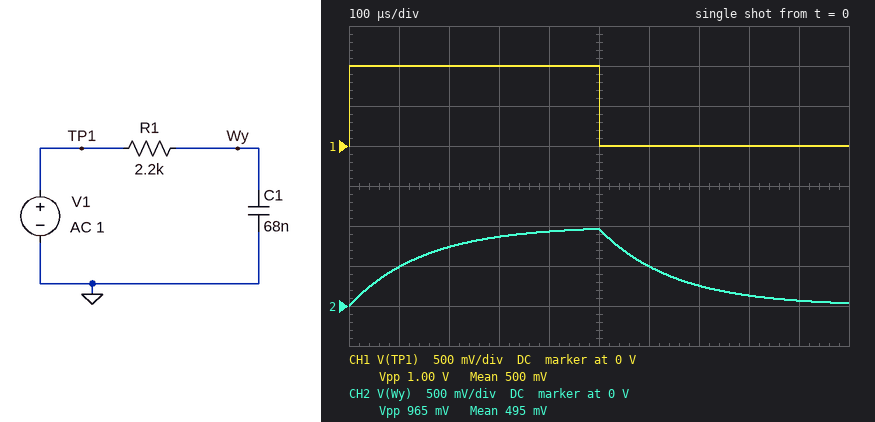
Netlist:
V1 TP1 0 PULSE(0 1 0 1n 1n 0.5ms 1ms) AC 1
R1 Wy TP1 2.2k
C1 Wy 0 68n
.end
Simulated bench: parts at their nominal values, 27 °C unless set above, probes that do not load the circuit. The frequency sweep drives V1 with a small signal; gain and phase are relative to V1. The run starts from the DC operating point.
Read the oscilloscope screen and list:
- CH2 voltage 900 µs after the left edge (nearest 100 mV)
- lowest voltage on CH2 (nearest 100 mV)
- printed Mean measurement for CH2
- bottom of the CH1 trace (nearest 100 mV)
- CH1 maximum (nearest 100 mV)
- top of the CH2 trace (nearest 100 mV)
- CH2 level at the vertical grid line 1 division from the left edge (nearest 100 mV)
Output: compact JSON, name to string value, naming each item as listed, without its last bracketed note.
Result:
{"CH2 voltage 900 µs after the left edge": "100 mV", "lowest voltage on CH2": "0 V", "printed Mean measurement for CH2": "495 mV", "bottom of the CH1 trace": "0 V", "CH1 maximum": "1.0 V", "top of the CH2 trace": "1.0 V", "CH2 level at the vertical grid line 1 division from the left edge": "500 mV"}
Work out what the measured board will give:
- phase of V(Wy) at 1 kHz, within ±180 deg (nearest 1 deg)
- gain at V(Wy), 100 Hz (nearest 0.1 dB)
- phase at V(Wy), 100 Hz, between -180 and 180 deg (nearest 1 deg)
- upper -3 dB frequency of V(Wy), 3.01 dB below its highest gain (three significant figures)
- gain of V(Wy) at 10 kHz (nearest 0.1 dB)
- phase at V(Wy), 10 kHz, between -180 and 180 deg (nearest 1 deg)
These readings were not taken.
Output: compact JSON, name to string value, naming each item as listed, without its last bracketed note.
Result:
{"phase of V(Wy) at 1 kHz, within ±180 deg": "-43 deg", "gain at V(Wy), 100 Hz": "0 dB", "phase at V(Wy), 100 Hz, between -180 and 180 deg": "-5 deg", "upper -3 dB frequency of V(Wy), 3.01 dB below its highest gain": "1.06 kHz", "gain of V(Wy) at 10 kHz": "-19.5 dB", "phase at V(Wy), 10 kHz, between -180 and 180 deg": "-84 deg"}
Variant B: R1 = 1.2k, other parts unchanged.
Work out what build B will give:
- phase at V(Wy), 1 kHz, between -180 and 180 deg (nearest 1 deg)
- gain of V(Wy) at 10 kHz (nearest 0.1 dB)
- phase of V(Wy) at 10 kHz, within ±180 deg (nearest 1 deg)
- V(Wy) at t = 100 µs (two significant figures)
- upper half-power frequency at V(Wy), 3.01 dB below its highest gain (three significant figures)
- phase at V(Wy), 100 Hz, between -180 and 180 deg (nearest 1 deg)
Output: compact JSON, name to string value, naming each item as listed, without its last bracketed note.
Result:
{"phase at V(Wy), 1 kHz, between -180 and 180 deg": "-27 deg", "gain of V(Wy) at 10 kHz": "-14.4 dB", "phase of V(Wy) at 10 kHz, within ±180 deg": "-79 deg", "V(Wy) at t = 100 µs": "710 mV", "upper half-power frequency at V(Wy), 3.01 dB below its highest gain": "1.95 kHz", "phase at V(Wy), 100 Hz, between -180 and 180 deg": "-3 deg"}
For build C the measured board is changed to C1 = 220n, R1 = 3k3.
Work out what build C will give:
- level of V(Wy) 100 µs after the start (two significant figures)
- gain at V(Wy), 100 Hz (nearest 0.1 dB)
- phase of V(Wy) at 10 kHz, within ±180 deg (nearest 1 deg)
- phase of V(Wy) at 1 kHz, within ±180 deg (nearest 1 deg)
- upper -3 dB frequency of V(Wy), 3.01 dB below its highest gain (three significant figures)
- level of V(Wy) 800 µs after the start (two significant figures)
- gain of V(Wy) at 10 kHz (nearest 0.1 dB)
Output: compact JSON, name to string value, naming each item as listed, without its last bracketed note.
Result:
{"level of V(Wy) 100 µs after the start": "130 mV", "gain at V(Wy), 100 Hz": "-0.8 dB", "phase of V(Wy) at 10 kHz, within ±180 deg": "-89 deg", "phase of V(Wy) at 1 kHz, within ±180 deg": "-78 deg", "upper -3 dB frequency of V(Wy), 3.01 dB below its highest gain": "219 Hz", "level of V(Wy) 800 µs after the start": "330 mV", "gain of V(Wy) at 10 kHz": "-33.2 dB"}
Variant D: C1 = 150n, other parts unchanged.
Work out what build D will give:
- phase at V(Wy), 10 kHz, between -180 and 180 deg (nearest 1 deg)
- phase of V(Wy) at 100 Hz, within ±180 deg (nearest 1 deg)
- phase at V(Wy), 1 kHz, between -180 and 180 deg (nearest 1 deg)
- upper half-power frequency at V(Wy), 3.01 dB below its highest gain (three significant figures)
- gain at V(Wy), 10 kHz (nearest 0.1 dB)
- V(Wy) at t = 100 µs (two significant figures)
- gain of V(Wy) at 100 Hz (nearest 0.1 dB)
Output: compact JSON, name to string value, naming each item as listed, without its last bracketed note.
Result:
{"phase at V(Wy), 10 kHz, between -180 and 180 deg": "-87 deg", "phase of V(Wy) at 100 Hz, within ±180 deg": "-12 deg", "phase at V(Wy), 1 kHz, between -180 and 180 deg": "-64 deg", "upper half-power frequency at V(Wy), 3.01 dB below its highest gain": "482 Hz", "gain at V(Wy), 10 kHz": "-26.3 dB", "V(Wy) at t = 100 µs": "260 mV", "gain of V(Wy) at 100 Hz": "-0.2 dB"}
